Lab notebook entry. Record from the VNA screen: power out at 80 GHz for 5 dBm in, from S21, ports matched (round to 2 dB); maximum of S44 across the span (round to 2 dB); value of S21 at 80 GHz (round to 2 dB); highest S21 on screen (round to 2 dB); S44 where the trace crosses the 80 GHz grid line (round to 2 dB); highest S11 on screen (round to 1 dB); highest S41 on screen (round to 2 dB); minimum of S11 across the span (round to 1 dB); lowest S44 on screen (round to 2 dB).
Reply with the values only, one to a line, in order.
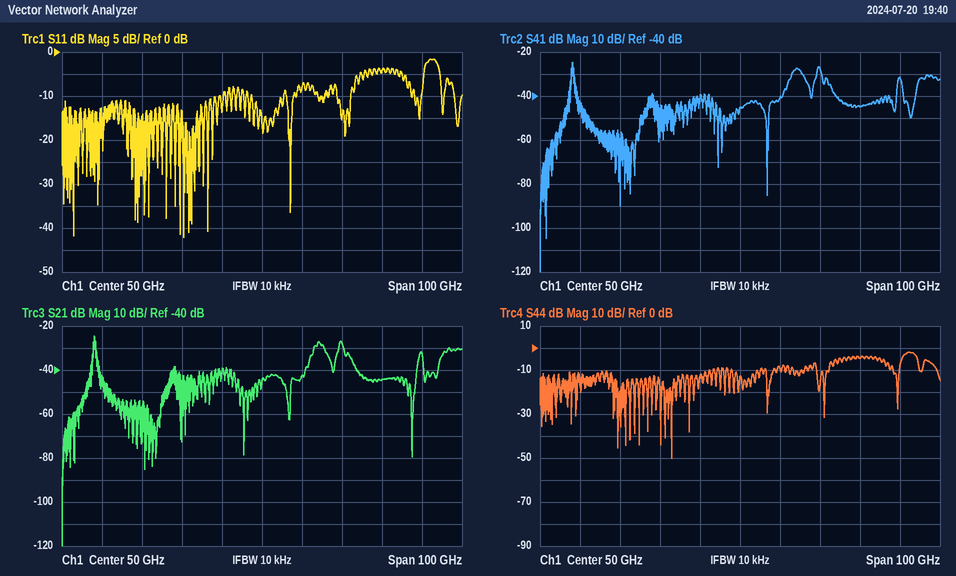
-40 dBm
-2 dB
-44 dB
-24 dB
-4 dB
-2 dB
-24 dB
-42 dB
-50 dB
